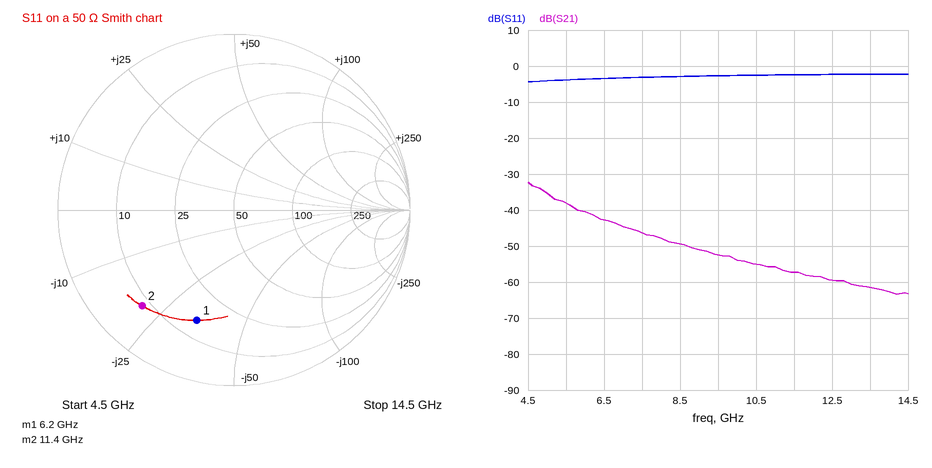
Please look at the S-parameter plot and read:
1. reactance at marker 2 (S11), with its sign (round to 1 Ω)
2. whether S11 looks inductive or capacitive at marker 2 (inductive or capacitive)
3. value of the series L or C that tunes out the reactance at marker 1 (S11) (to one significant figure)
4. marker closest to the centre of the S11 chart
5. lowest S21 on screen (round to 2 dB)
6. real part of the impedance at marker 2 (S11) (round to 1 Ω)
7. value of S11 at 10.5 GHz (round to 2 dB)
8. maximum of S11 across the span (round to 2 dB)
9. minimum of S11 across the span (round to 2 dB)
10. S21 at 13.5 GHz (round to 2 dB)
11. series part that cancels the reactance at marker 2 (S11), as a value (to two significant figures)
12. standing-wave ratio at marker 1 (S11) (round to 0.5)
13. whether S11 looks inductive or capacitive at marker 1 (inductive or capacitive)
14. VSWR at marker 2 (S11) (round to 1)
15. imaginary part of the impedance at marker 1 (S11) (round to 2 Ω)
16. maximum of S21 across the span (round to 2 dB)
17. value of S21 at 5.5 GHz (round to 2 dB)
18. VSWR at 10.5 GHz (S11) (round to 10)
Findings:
-21 Ω
capacitive
900 pH
marker 1
-64 dB
8 Ω
-2 dB
-2 dB
-4 dB
-62 dB
290 pH
5.0
capacitive
7
-34 Ω
-32 dB
-38 dB
10
